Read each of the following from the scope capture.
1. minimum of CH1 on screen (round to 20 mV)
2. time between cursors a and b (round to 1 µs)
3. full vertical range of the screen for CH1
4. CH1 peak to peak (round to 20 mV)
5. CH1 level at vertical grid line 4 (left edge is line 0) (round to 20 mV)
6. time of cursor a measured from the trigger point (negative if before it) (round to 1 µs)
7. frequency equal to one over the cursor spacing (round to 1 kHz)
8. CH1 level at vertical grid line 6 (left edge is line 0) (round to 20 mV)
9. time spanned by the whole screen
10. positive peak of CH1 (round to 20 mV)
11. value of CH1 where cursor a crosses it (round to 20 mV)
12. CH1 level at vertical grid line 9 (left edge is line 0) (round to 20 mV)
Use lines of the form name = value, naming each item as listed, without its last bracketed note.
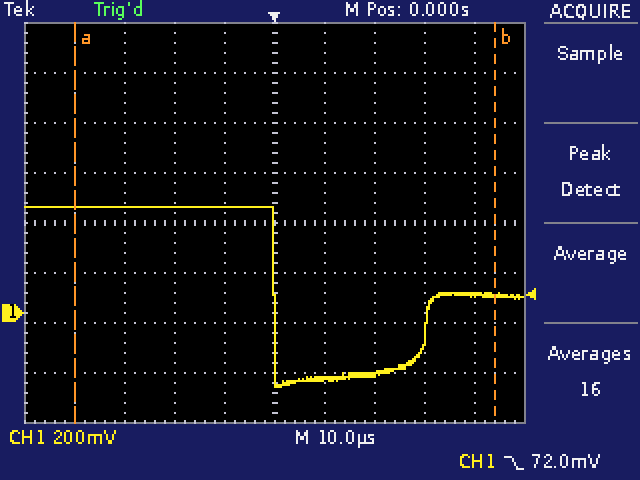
minimum of CH1 on screen = -300 mV
time between cursors a and b = 84 µs
full vertical range of the screen for CH1 = 1.6 V
CH1 peak to peak = 720 mV
CH1 level at vertical grid line 4 (left edge is line 0) = 420 mV
time of cursor a measured from the trigger point (negative if before it) = -40 µs
frequency equal to one over the cursor spacing = 12 kHz
CH1 level at vertical grid line 6 (left edge is line 0) = -260 mV
time spanned by the whole screen = 100 µs
positive peak of CH1 = 420 mV
value of CH1 where cursor a crosses it = 420 mV
CH1 level at vertical grid line 9 (left edge is line 0) = 80 mV
